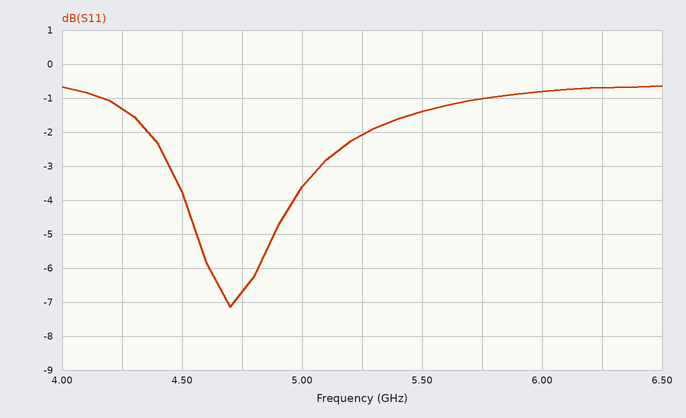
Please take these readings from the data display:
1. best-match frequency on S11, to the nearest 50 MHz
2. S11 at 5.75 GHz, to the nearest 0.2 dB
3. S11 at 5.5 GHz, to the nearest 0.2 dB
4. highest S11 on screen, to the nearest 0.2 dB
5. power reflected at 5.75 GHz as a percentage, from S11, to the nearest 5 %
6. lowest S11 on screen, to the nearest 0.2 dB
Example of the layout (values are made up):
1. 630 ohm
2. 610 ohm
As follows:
1. 4.70 GHz
2. -1.0 dB
3. -1.4 dB
4. -0.6 dB
5. 80 %
6. -7.2 dB
